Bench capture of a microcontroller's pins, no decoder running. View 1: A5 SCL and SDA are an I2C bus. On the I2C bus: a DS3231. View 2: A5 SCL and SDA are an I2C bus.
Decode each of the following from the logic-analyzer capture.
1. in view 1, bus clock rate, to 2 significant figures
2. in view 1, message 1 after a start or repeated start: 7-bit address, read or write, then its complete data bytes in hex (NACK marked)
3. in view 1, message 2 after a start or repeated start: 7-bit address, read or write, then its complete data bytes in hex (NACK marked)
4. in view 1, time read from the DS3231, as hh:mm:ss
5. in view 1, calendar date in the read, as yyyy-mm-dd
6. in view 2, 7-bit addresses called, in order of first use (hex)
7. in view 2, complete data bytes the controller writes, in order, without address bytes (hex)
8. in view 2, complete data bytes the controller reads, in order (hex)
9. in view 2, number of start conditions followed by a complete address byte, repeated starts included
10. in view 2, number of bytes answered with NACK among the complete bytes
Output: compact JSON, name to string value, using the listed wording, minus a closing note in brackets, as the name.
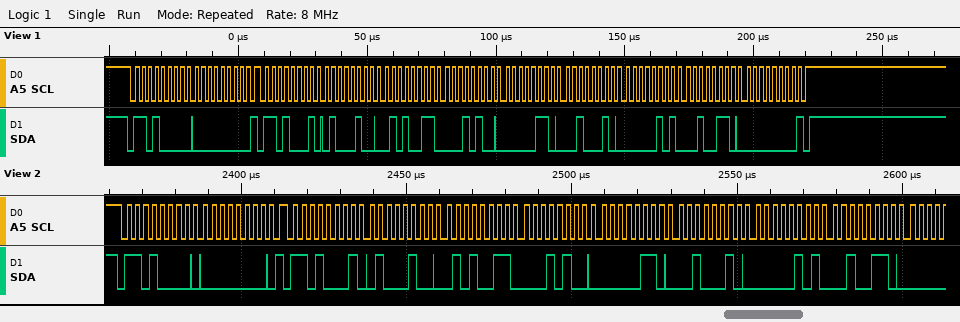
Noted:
{"in view 1, bus clock rate, to 2 significant figures": "400 kHz", "in view 1, message 1 after a start or repeated start: 7-bit address, read or write, then its complete data bytes in hex": "0x68 write: 00", "in view 1, message 2 after a start or repeated start: 7-bit address, read or write, then its complete data bytes in hex": "0x68 read: 44 53 14 06 22 05 26 00 NACK", "in view 1, time read from the DS3231, as hh:mm:ss": "14:53:44", "in view 1, calendar date in the read, as yyyy-mm-dd": "2026-05-22", "in view 2, 7-bit addresses called, in order of first use": "0x68", "in view 2, complete data bytes the controller writes, in order, without address bytes": "00", "in view 2, complete data bytes the controller reads, in order": "44 53 14 06 22 05 26", "in view 2, number of start conditions followed by a complete address byte, repeated starts included": "2", "in view 2, number of bytes answered with NACK among the complete bytes": "0"}
